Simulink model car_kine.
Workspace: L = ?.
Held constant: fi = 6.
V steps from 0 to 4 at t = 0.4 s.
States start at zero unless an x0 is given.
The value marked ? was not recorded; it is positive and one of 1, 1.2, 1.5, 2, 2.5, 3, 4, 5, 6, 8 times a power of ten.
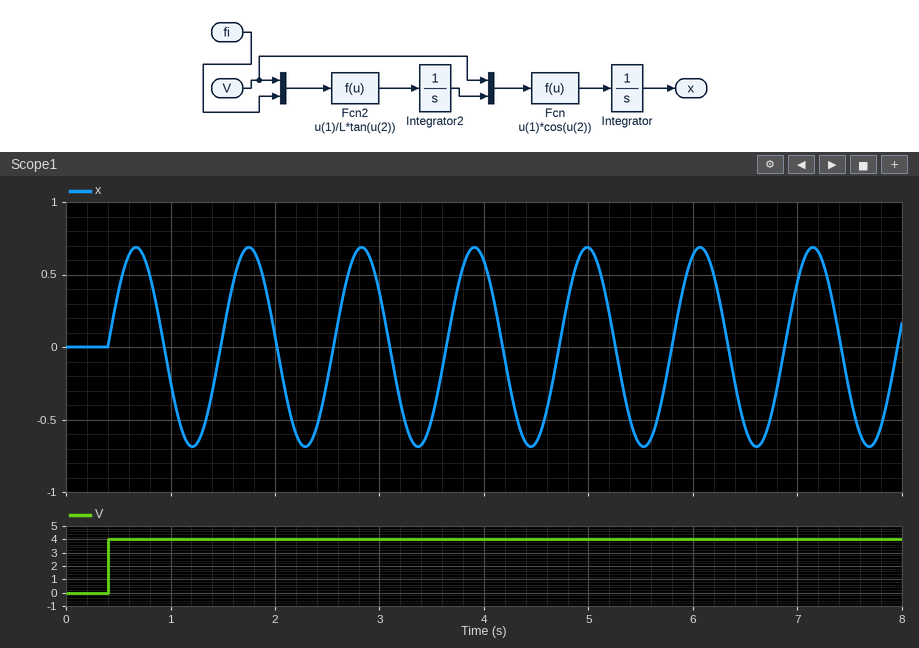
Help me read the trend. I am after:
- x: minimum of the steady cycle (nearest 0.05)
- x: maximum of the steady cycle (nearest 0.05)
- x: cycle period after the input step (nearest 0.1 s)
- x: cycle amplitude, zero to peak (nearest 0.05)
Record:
-0.70
0.70
1.1 s
0.70
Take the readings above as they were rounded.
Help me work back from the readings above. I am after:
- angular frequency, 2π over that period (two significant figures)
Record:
5.7 rad/s
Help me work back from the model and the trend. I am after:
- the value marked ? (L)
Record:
0.2
